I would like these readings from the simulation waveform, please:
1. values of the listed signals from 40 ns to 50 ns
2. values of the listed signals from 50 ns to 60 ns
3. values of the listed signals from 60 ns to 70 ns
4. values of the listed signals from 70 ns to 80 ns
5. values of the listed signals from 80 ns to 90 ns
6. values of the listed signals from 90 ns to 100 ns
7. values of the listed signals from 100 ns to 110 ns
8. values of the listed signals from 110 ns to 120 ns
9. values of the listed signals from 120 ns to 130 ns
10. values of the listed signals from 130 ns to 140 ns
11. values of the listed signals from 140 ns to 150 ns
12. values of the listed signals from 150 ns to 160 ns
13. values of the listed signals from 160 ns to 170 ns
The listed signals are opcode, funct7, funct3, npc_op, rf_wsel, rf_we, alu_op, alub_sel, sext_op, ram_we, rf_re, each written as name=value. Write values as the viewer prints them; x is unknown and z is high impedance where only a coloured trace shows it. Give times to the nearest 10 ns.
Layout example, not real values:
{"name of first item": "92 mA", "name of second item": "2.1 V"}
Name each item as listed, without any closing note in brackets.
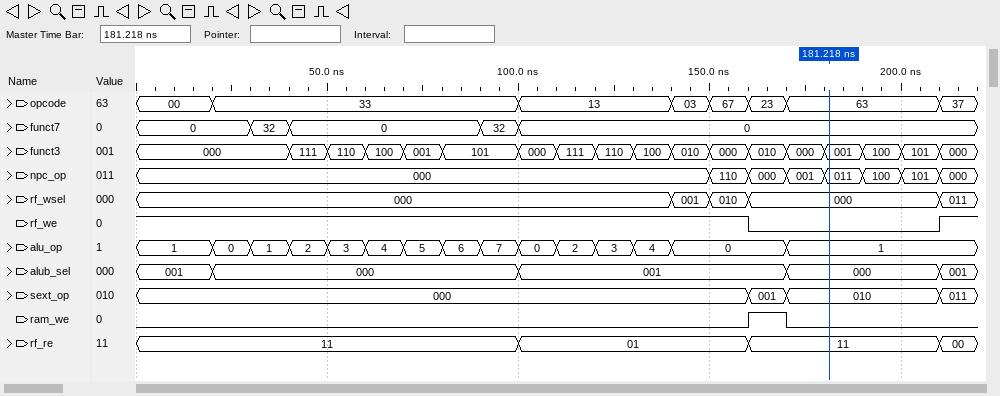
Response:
{"values of the listed signals from 40 ns to 50 ns": "opcode=33, funct7=0, funct3=111, npc_op=000, rf_wsel=000, rf_we=1, alu_op=2, alub_sel=000, sext_op=000, ram_we=0, rf_re=11", "values of the listed signals from 50 ns to 60 ns": "opcode=33, funct7=0, funct3=110, npc_op=000, rf_wsel=000, rf_we=1, alu_op=3, alub_sel=000, sext_op=000, ram_we=0, rf_re=11", "values of the listed signals from 60 ns to 70 ns": "opcode=33, funct7=0, funct3=100, npc_op=000, rf_wsel=000, rf_we=1, alu_op=4, alub_sel=000, sext_op=000, ram_we=0, rf_re=11", "values of the listed signals from 70 ns to 80 ns": "opcode=33, funct7=0, funct3=001, npc_op=000, rf_wsel=000, rf_we=1, alu_op=5, alub_sel=000, sext_op=000, ram_we=0, rf_re=11", "values of the listed signals from 80 ns to 90 ns": "opcode=33, funct7=0, funct3=101, npc_op=000, rf_wsel=000, rf_we=1, alu_op=6, alub_sel=000, sext_op=000, ram_we=0, rf_re=11", "values of the listed signals from 90 ns to 100 ns": "opcode=33, funct7=32, funct3=101, npc_op=000, rf_wsel=000, rf_we=1, alu_op=7, alub_sel=000, sext_op=000, ram_we=0, rf_re=11", "values of the listed signals from 100 ns to 110 ns": "opcode=13, funct7=0, funct3=000, npc_op=000, rf_wsel=000, rf_we=1, alu_op=0, alub_sel=001, sext_op=000, ram_we=0, rf_re=01", "values of the listed signals from 110 ns to 120 ns": "opcode=13, funct7=0, funct3=111, npc_op=000, rf_wsel=000, rf_we=1, alu_op=2, alub_sel=001, sext_op=000, ram_we=0, rf_re=01", "values of the listed signals from 120 ns to 130 ns": "opcode=13, funct7=0, funct3=110, npc_op=000, rf_wsel=000, rf_we=1, alu_op=3, alub_sel=001, sext_op=000, ram_we=0, rf_re=01", "values of the listed signals from 130 ns to 140 ns": "opcode=13, funct7=0, funct3=100, npc_op=000, rf_wsel=000, rf_we=1, alu_op=4, alub_sel=001, sext_op=000, ram_we=0, rf_re=01", "values of the listed signals from 140 ns to 150 ns": "opcode=03, funct7=0, funct3=010, npc_op=000, rf_wsel=001, rf_we=1, alu_op=0, alub_sel=001, sext_op=000, ram_we=0, rf_re=01", "values of the listed signals from 150 ns to 160 ns": "opcode=67, funct7=0, funct3=000, npc_op=110, rf_wsel=010, rf_we=1, alu_op=0, alub_sel=001, sext_op=000, ram_we=0, rf_re=01", "values of the listed signals from 160 ns to 170 ns": "opcode=23, funct7=0, funct3=010, npc_op=000, rf_wsel=000, rf_we=0, alu_op=0, alub_sel=001, sext_op=001, ram_we=1, rf_re=11"}
